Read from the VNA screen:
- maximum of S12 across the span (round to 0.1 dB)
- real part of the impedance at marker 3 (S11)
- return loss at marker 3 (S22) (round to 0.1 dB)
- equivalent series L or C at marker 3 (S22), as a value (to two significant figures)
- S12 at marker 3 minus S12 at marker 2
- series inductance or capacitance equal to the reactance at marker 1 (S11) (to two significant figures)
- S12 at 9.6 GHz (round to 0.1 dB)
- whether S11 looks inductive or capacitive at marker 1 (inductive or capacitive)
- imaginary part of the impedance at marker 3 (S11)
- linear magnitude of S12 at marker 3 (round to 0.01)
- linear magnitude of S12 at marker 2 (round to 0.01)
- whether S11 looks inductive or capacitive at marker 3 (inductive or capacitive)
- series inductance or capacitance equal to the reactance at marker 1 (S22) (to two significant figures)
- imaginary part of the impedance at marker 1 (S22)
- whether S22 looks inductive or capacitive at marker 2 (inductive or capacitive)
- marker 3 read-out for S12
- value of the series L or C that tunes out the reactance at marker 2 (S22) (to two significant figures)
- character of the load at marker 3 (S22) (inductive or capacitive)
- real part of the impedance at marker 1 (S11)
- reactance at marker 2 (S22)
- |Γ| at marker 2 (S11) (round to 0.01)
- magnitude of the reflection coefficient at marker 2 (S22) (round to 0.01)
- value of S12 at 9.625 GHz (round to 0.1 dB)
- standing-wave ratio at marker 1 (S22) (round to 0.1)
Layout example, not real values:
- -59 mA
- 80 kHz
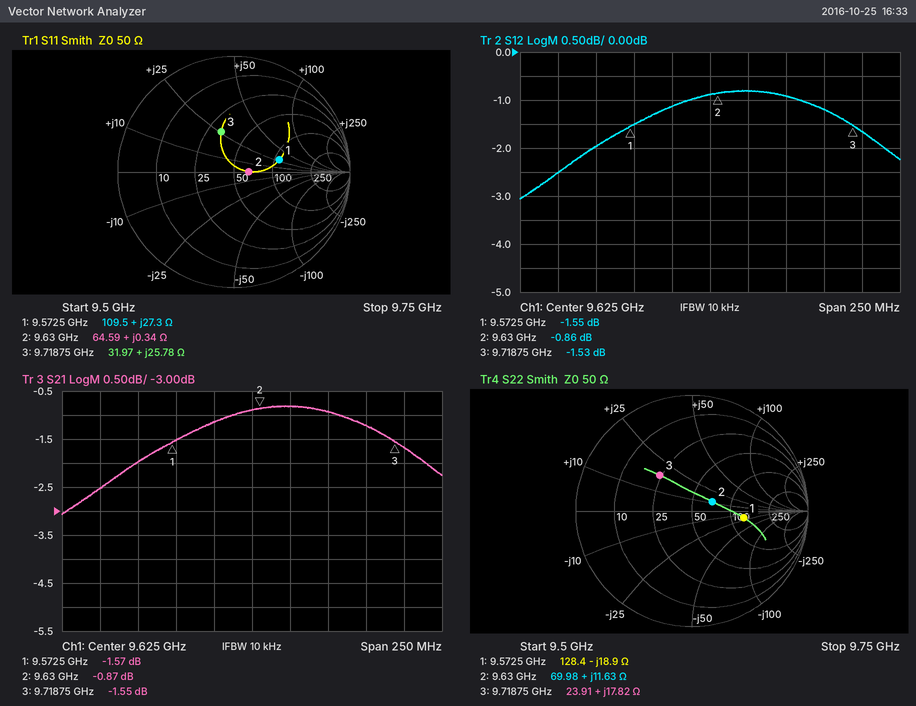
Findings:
- -0.8 dB
- 31.97 Ω
- 7.6 dB
- 290 pH
- -0.67 dB
- 450 pH
- -1.1 dB
- inductive
- +25.78 Ω
- 0.84
- 0.91
- inductive
- 880 fF
- -18.9 Ω
- inductive
- -1.53 dB
- 1.4 pF
- inductive
- 109.5 Ω
- +11.63 Ω
- 0.13
- 0.19
- -0.9 dB
- 2.6
